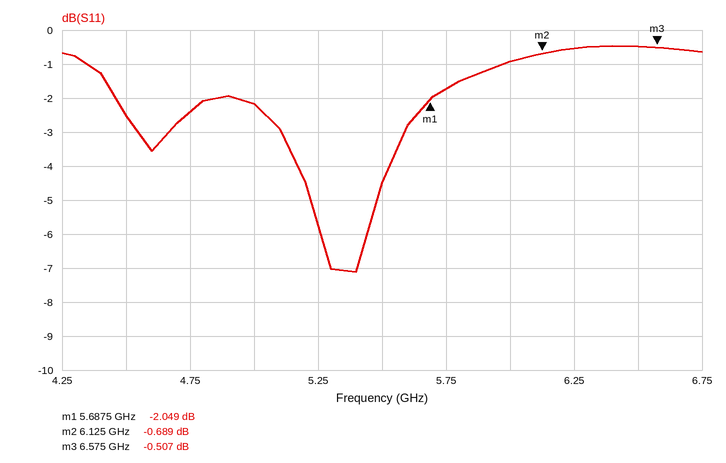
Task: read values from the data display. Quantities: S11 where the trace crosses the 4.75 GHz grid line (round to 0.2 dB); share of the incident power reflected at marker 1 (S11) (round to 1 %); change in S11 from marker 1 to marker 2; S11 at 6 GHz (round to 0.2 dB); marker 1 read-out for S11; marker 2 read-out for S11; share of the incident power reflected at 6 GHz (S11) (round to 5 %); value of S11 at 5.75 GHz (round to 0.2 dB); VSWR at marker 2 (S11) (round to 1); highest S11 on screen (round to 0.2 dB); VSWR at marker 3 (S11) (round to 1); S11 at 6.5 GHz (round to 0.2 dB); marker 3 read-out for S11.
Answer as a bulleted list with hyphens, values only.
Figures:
- -2.4 dB
- 62 %
- 1.360 dB
- -1.0 dB
- -2.049 dB
- -0.689 dB
- 80 %
- -1.8 dB
- 25
- -0.4 dB
- 34
- -0.4 dB
- -0.507 dB
